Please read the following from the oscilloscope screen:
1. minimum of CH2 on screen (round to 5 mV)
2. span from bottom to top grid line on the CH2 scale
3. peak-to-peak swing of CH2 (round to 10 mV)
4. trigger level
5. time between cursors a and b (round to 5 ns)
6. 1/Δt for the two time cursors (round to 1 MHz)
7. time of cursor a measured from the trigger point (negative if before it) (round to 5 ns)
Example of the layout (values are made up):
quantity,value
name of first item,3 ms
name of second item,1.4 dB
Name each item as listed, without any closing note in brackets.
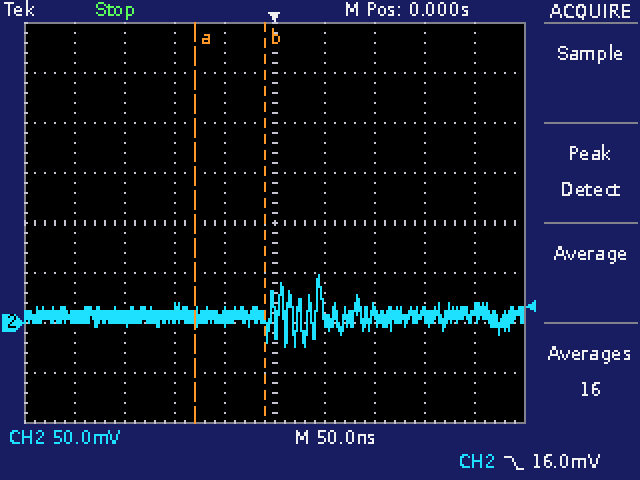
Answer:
quantity,value
minimum of CH2 on screen,-25 mV
span from bottom to top grid line on the CH2 scale,400 mV
peak-to-peak swing of CH2,70 mV
trigger level,16.0 mV
time between cursors a and b,70 ns
1/Δt for the two time cursors,14 MHz
time of cursor a measured from the trigger point (negative if before it),-80 ns
